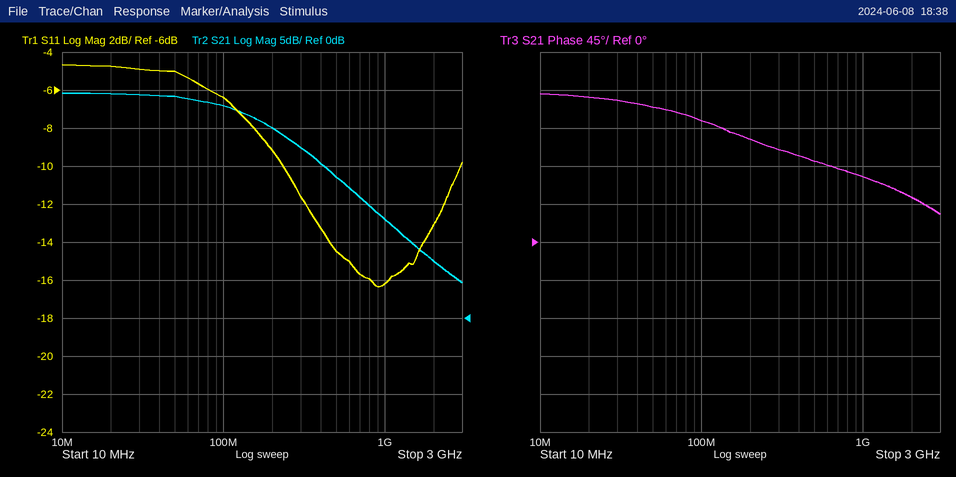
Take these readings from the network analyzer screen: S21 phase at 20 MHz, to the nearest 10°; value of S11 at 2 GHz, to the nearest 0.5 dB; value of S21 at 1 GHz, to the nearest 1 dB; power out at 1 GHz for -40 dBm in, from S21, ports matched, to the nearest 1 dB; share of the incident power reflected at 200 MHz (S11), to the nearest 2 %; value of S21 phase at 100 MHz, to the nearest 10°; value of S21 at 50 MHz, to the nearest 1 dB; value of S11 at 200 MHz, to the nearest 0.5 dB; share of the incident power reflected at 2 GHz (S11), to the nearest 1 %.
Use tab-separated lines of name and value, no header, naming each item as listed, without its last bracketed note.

S21 phase at 20 MHz, to the nearest 10°	170°
value of S11 at 2 GHz, to the nearest 0.5 dB	-13.0 dB
value of S21 at 1 GHz, to the nearest 1 dB	13 dB
power out at 1 GHz for -40 dBm in, from S21, ports matched, to the nearest 1 dB	-27 dBm
share of the incident power reflected at 200 MHz (S11), to the nearest 2 %	12 %
value of S21 phase at 100 MHz, to the nearest 10°	140°
value of S21 at 50 MHz, to the nearest 1 dB	29 dB
value of S11 at 200 MHz, to the nearest 0.5 dB	-9.0 dB
share of the incident power reflected at 2 GHz (S11), to the nearest 1 %	5 %
